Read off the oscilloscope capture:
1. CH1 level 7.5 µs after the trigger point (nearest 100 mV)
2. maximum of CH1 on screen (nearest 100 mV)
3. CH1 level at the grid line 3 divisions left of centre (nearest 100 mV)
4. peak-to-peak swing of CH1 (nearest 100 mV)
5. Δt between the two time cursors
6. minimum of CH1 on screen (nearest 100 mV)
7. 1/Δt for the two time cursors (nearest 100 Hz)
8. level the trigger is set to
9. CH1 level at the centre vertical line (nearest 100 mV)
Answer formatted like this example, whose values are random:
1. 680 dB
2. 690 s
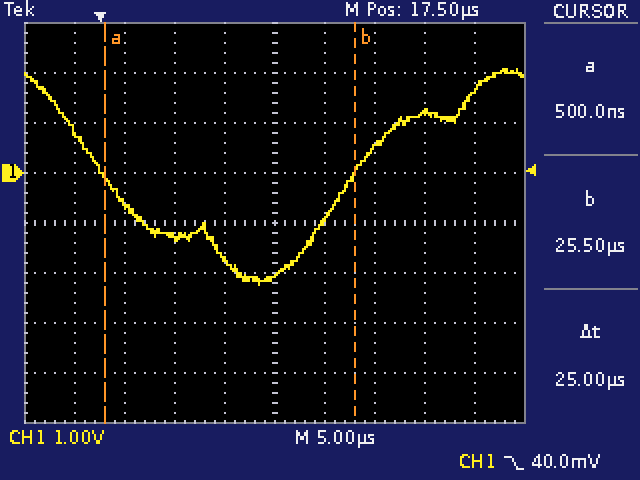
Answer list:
1. -1.3 V
2. 2.1 V
3. -600 mV
4. 4.3 V
5. 25 µs
6. -2.2 V
7. 40.0 kHz
8. 40.0 mV
9. -2.1 V
